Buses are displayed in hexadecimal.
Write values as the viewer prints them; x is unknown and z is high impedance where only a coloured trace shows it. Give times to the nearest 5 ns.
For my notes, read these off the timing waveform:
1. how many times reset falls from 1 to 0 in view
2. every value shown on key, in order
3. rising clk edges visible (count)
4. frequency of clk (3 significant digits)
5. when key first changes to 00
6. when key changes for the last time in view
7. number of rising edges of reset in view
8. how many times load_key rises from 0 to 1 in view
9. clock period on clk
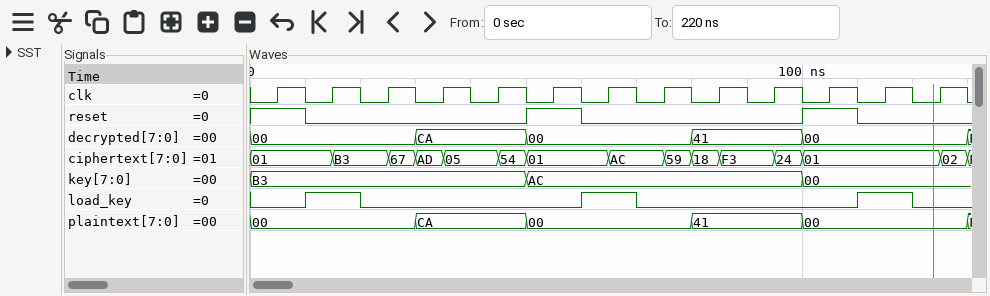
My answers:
3
B3, AC, 00
13
100 MHz
100 ns
100 ns
2
3
10 ns
